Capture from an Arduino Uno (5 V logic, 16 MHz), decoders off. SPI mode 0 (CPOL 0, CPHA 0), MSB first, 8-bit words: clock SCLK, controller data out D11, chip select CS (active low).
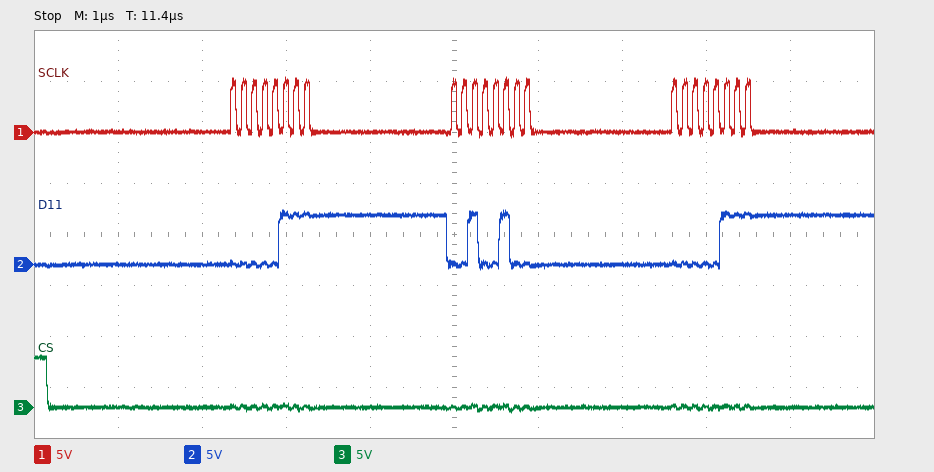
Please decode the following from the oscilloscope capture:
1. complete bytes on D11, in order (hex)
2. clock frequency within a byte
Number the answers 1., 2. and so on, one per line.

1. 07 24 07
2. 8 MHz
